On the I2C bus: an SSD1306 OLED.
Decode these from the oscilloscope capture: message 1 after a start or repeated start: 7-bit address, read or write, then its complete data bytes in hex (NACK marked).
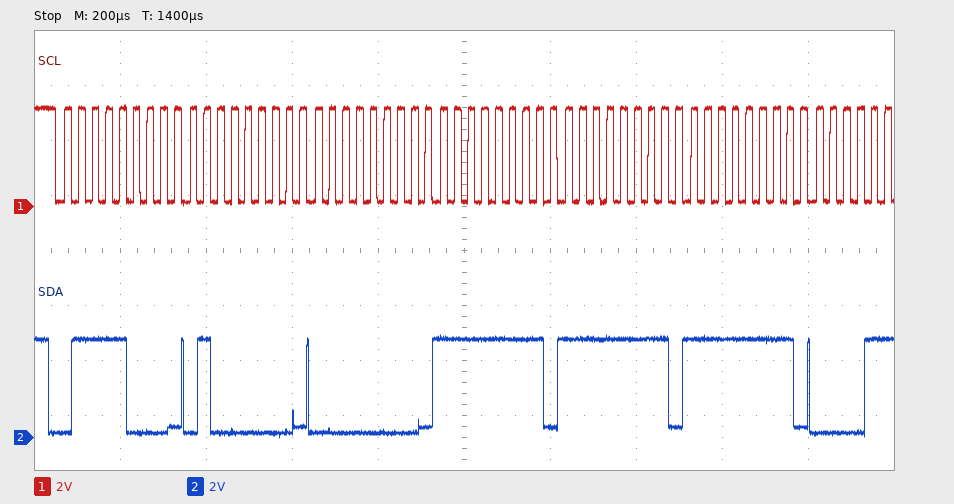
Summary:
0x3C write: 40 00 FF FF FF
